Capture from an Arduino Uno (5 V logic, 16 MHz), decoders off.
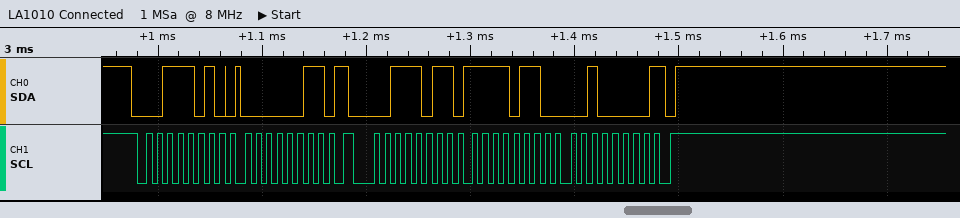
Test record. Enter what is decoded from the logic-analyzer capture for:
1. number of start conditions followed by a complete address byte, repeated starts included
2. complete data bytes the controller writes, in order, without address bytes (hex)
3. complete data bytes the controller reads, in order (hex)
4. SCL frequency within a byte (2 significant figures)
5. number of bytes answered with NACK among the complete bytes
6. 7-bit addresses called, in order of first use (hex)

2
03
F6 20
100 kHz
1
0x1D
